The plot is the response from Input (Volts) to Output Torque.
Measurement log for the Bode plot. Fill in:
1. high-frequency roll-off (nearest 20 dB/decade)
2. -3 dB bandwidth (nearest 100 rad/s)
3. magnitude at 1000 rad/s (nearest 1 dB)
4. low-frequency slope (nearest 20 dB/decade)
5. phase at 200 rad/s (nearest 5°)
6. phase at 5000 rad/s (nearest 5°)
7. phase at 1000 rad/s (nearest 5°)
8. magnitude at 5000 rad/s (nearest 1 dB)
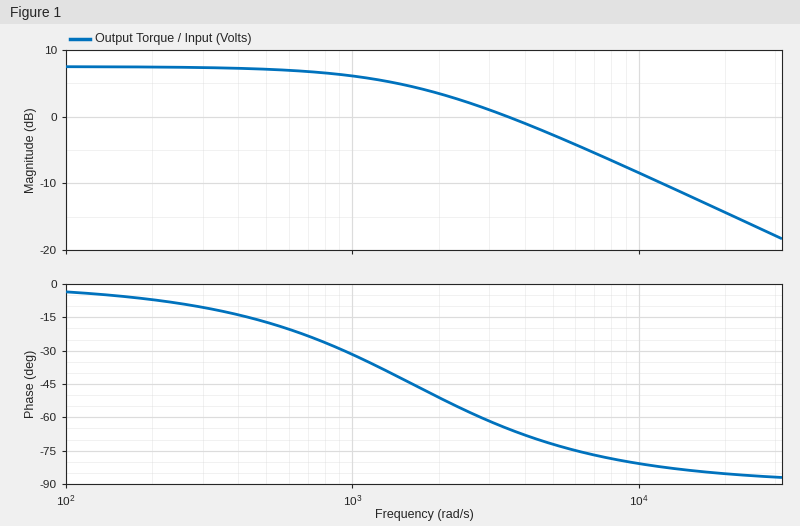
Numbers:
-20 dB/decade
1600 rad/s
6 dB
0 dB/decade
-5°
-70°
-30°
-3 dB
